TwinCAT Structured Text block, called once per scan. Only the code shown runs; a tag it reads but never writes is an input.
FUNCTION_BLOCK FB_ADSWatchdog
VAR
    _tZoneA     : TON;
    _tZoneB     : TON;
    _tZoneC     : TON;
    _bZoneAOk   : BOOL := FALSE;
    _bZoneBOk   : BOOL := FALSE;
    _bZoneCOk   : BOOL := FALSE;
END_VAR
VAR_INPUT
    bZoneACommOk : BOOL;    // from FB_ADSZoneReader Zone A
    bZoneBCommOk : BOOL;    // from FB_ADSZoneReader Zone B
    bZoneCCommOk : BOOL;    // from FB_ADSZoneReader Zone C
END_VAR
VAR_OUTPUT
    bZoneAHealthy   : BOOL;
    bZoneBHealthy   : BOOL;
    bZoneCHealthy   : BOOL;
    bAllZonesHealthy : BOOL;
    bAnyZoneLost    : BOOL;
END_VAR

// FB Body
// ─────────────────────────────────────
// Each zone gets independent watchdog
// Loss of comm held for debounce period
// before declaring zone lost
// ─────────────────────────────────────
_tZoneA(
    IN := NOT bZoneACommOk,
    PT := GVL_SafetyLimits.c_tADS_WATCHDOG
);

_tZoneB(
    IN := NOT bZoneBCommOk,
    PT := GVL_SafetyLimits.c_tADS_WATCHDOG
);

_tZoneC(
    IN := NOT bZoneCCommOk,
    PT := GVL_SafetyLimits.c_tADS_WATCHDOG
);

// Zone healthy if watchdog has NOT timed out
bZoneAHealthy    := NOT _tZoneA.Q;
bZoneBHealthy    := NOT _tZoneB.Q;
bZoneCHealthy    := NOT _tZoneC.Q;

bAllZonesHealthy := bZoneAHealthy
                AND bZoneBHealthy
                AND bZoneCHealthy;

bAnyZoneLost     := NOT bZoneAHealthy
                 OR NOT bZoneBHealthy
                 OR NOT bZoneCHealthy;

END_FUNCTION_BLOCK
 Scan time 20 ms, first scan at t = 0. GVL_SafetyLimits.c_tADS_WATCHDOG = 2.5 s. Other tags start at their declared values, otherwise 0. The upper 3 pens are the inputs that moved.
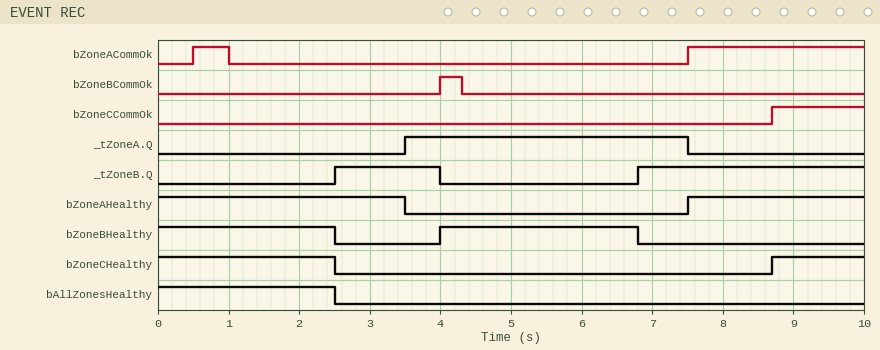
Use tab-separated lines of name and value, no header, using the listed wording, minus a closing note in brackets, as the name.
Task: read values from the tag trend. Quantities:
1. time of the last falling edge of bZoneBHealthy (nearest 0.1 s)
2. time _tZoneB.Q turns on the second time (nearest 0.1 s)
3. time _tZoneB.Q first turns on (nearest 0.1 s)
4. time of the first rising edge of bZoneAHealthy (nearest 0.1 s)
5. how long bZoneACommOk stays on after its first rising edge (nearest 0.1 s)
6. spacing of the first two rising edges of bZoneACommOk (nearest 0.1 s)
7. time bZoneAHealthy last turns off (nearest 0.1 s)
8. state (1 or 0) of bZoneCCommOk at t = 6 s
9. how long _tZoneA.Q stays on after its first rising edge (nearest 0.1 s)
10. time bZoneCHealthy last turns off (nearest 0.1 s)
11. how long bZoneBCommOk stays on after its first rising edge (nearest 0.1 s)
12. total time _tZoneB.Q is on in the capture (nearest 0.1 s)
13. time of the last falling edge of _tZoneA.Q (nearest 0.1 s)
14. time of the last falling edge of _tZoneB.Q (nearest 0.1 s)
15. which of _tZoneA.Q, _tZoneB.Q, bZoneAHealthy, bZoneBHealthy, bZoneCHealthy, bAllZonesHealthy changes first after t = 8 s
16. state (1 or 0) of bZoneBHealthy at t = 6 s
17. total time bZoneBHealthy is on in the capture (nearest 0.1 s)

time of the last falling edge of bZoneBHealthy	6.8 s
time _tZoneB.Q turns on the second time	6.8 s
time _tZoneB.Q first turns on	2.5 s
time of the first rising edge of bZoneAHealthy	7.5 s
how long bZoneACommOk stays on after its first rising edge	0.5 s
spacing of the first two rising edges of bZoneACommOk	7.0 s
time bZoneAHealthy last turns off	3.5 s
state (1 or 0) of bZoneCCommOk at t = 6 s	0
how long _tZoneA.Q stays on after its first rising edge	4.0 s
time bZoneCHealthy last turns off	2.5 s
how long bZoneBCommOk stays on after its first rising edge	0.3 s
total time _tZoneB.Q is on in the capture	4.7 s
time of the last falling edge of _tZoneA.Q	7.5 s
time of the last falling edge of _tZoneB.Q	4.0 s
which of _tZoneA.Q, _tZoneB.Q, bZoneAHealthy, bZoneBHealthy, bZoneCHealthy, bAllZonesHealthy changes first after t = 8 s	bZoneCHealthy
state (1 or 0) of bZoneBHealthy at t = 6 s	1
total time bZoneBHealthy is on in the capture	5.3 s
